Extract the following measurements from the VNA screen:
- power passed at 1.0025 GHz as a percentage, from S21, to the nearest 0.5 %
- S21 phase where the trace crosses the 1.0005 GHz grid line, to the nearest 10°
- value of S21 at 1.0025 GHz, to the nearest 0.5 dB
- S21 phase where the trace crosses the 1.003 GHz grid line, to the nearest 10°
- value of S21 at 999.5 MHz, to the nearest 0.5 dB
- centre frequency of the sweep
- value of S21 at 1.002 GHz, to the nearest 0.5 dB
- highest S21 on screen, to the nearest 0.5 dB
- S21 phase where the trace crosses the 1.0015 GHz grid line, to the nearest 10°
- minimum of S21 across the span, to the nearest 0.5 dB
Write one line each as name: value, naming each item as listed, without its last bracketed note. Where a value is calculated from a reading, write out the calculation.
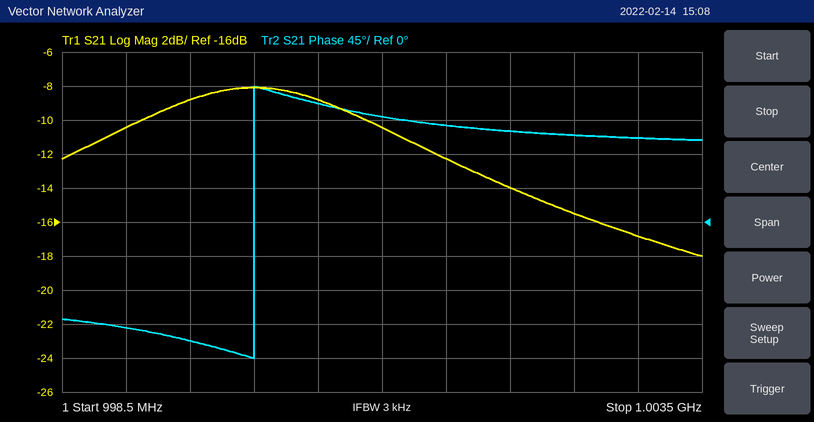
power passed at 1.0025 GHz as a percentage, from S21, to the nearest 0.5 %: 10^(-15.5/10) ≈ 2.82 %, so 3.0 % to the nearest 0.5 %
S21 phase where the trace crosses the 1.0005 GHz grid line, to the nearest 10°: 160°
value of S21 at 1.0025 GHz, to the nearest 0.5 dB: -15.5 dB
S21 phase where the trace crosses the 1.003 GHz grid line, to the nearest 10°: 110°
value of S21 at 999.5 MHz, to the nearest 0.5 dB: -9.0 dB
centre frequency of the sweep: 1.001 GHz
value of S21 at 1.002 GHz, to the nearest 0.5 dB: -14.0 dB
highest S21 on screen, to the nearest 0.5 dB: -8.0 dB
S21 phase where the trace crosses the 1.0015 GHz grid line, to the nearest 10°: 130°
minimum of S21 across the span, to the nearest 0.5 dB: -18.0 dB
